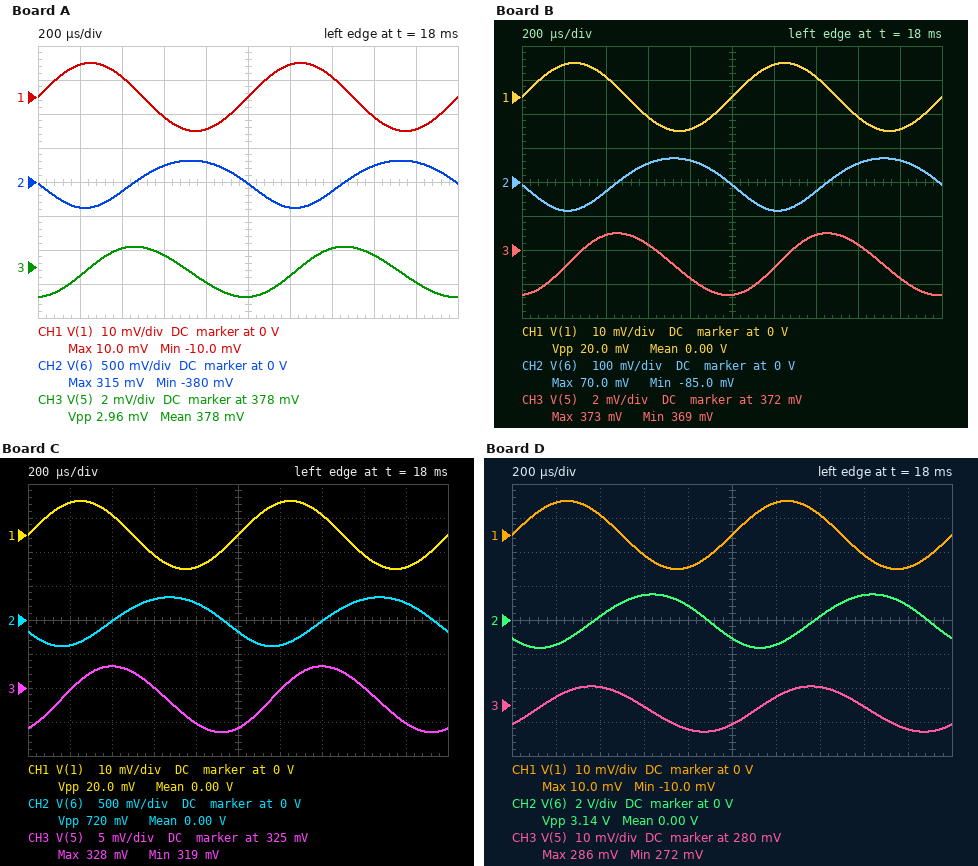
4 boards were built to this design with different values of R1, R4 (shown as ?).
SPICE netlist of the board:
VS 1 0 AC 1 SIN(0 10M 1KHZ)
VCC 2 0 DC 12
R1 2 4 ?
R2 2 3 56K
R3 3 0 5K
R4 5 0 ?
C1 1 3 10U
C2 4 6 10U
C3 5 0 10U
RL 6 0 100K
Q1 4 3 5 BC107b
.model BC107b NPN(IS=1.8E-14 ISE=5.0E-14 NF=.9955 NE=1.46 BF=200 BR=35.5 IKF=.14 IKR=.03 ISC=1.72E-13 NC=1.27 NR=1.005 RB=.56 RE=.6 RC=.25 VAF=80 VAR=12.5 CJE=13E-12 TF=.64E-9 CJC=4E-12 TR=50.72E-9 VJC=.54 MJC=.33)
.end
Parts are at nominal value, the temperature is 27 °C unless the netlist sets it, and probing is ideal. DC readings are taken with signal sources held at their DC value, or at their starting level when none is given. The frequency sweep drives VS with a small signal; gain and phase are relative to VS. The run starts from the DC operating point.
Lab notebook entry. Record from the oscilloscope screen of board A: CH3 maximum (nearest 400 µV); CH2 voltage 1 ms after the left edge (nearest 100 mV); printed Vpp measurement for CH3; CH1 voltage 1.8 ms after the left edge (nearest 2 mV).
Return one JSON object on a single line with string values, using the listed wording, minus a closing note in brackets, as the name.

{"CH3 maximum": "379.2 mV", "CH2 voltage 1 ms after the left edge": "0 V", "printed Vpp measurement for CH3": "2.96 mV", "CH1 voltage 1.8 ms after the left edge": "-10 mV"}
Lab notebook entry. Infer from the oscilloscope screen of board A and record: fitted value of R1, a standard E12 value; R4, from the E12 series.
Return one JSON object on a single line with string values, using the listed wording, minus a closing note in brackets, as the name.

{"fitted value of R1, a standard E12 value": "3.9 kΩ", "R4, from the E12 series": "1.5 kΩ"}
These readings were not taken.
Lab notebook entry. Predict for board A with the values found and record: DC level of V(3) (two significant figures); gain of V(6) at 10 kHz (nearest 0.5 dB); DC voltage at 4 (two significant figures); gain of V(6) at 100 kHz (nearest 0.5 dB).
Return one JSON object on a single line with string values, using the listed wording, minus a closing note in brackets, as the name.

{"DC level of V(3)": "980 mV", "gain of V(6) at 10 kHz": "31.0 dB", "DC voltage at 4": "11 V", "gain of V(6) at 100 kHz": "31.0 dB"}
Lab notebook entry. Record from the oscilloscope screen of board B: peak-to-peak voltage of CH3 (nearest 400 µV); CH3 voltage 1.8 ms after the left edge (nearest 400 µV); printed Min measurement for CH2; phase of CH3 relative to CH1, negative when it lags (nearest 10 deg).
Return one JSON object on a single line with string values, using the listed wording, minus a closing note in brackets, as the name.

{"peak-to-peak voltage of CH3": "3.6 mV", "CH3 voltage 1.8 ms after the left edge": "370.4 mV", "printed Min measurement for CH2": "-85.0 mV", "phase of CH3 relative to CH1, negative when it lags": "-80 deg"}
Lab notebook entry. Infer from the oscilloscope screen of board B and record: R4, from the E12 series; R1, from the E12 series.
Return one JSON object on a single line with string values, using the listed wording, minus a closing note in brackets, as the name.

{"R4, from the E12 series": "1.2 kΩ", "R1, from the E12 series": "680 Ω"}
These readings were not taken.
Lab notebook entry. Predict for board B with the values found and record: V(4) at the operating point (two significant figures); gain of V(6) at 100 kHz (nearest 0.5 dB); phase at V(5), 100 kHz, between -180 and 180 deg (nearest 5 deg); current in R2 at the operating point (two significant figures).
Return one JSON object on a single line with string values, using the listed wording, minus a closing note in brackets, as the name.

{"V(4) at the operating point": "12 V", "gain of V(6) at 100 kHz": "18.0 dB", "phase at V(5), 100 kHz, between -180 and 180 deg": "-90 deg", "current in R2 at the operating point": "200 µA"}
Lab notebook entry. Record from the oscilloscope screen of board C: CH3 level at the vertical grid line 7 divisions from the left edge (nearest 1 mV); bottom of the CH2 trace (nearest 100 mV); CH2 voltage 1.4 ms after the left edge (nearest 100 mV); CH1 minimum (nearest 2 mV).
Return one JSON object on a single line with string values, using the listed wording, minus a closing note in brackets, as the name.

{"CH3 level at the vertical grid line 7 divisions from the left edge": "328 mV", "bottom of the CH2 trace": "-400 mV", "CH2 voltage 1.4 ms after the left edge": "0 V", "CH1 minimum": "-10 mV"}
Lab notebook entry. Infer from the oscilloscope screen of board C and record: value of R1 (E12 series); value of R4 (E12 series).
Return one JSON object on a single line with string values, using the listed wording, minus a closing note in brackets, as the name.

{"value of R1": "1.2 kΩ", "value of R4": "330 Ω"}
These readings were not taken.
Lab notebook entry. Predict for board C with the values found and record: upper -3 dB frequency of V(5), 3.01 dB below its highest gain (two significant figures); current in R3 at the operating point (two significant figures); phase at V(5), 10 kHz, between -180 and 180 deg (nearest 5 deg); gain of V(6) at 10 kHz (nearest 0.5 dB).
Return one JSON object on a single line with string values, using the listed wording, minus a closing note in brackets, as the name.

{"upper -3 dB frequency of V(5), 3.01 dB below its highest gain": "640 Hz", "current in R3 at the operating point": "190 µA", "phase at V(5), 10 kHz, between -180 and 180 deg": "-85 deg", "gain of V(6) at 10 kHz": "32.5 dB"}
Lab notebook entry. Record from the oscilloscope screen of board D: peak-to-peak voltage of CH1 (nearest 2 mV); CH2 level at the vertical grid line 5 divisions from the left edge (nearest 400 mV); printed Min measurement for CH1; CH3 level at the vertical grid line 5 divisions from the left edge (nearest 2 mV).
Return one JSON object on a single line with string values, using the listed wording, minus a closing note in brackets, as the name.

{"peak-to-peak voltage of CH1": "20 mV", "CH2 level at the vertical grid line 5 divisions from the left edge": "-1.2 V", "printed Min measurement for CH1": "-10.0 mV", "CH3 level at the vertical grid line 5 divisions from the left edge": "274 mV"}
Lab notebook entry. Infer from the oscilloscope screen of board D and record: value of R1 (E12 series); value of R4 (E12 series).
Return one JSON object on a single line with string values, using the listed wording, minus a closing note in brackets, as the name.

{"value of R1": "3.9 kΩ", "value of R4": "150 Ω"}
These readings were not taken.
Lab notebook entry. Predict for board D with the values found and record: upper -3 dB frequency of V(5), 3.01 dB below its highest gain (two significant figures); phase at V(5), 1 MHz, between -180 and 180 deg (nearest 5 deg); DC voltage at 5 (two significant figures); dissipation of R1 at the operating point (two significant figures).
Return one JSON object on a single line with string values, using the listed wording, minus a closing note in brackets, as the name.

{"upper -3 dB frequency of V(5), 3.01 dB below its highest gain": "1.1 kHz", "phase at V(5), 1 MHz, between -180 and 180 deg": "-90 deg", "DC voltage at 5": "280 mV", "dissipation of R1 at the operating point": "13 mW"}
